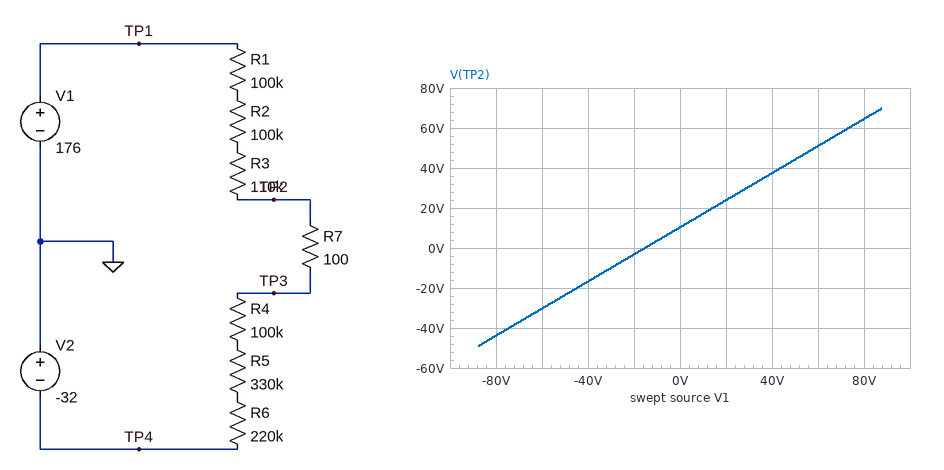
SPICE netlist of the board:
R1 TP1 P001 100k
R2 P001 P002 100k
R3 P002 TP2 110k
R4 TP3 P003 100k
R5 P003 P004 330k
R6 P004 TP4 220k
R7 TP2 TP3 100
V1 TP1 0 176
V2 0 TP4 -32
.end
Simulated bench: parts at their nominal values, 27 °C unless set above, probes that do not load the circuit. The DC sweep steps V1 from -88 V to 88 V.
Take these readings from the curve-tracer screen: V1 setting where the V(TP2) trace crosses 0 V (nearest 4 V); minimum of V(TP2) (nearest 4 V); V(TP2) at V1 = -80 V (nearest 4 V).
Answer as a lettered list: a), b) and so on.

a) -16 V
b) -48 V
c) -44 V
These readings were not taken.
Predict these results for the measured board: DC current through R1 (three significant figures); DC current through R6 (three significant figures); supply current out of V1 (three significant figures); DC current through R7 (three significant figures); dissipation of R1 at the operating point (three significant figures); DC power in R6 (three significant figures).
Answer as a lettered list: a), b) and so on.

a) 150 µA
b) 150 µA
c) 150 µA
d) 150 µA
e) 2.25 mW
f) 4.95 mW
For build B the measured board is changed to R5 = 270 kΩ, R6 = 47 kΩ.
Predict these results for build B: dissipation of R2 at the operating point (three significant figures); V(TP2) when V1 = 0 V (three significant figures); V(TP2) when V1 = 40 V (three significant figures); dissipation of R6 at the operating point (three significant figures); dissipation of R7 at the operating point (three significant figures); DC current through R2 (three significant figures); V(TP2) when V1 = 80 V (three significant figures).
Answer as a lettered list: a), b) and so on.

a) 3.92 mW
b) 13.6 V
c) 36.6 V
d) 1.84 mW
e) 3.92 µW
f) 198 µA
g) 59.5 V
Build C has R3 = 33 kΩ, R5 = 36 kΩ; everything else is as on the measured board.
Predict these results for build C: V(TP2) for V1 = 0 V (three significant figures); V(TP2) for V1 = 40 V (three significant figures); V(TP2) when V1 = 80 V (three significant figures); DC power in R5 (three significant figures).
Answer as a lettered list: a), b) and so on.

a) 12.7 V
b) 36.8 V
c) 61.0 V
d) 2.15 mW
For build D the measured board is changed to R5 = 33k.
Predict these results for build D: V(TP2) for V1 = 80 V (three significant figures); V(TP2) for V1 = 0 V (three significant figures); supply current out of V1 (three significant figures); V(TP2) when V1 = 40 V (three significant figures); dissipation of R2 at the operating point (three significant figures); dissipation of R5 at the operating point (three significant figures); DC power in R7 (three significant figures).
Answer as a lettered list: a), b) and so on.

a) 57.6 V
b) 15.0 V
c) 217 µA
d) 36.3 V
e) 4.72 mW
f) 1.56 mW
g) 4.72 µW
